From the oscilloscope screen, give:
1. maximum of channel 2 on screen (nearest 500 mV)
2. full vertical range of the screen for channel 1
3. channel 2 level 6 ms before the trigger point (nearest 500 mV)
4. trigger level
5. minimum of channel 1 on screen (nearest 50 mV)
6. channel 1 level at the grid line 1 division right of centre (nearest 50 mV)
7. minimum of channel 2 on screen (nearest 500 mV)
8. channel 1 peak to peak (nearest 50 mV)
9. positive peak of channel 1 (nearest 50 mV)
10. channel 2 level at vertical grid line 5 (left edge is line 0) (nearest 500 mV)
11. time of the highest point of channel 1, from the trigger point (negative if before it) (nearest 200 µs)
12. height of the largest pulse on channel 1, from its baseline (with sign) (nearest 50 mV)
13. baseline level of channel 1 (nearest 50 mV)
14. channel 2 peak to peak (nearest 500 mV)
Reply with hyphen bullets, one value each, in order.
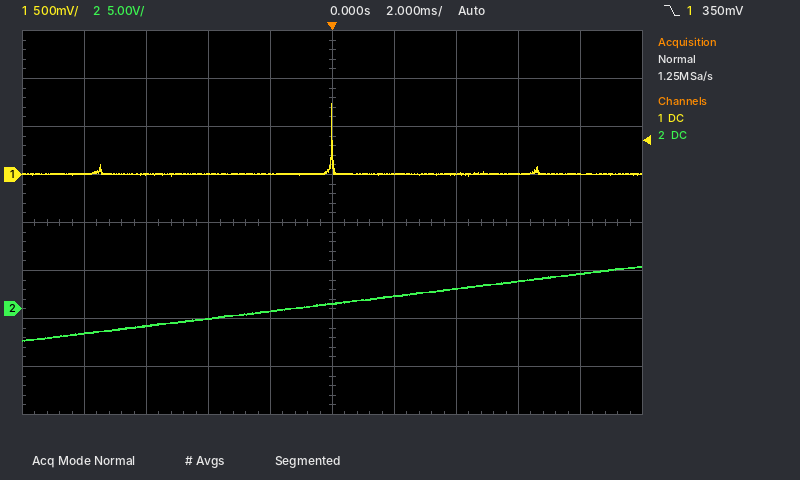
- 4.5 V
- 4 V
- -2.0 V
- 350 mV
- 0 mV
- 0 mV
- -3.5 V
- 750 mV
- 750 mV
- 500 mV
- 0.0 ms
- +750 mV
- 0 mV
- 8.0 V
